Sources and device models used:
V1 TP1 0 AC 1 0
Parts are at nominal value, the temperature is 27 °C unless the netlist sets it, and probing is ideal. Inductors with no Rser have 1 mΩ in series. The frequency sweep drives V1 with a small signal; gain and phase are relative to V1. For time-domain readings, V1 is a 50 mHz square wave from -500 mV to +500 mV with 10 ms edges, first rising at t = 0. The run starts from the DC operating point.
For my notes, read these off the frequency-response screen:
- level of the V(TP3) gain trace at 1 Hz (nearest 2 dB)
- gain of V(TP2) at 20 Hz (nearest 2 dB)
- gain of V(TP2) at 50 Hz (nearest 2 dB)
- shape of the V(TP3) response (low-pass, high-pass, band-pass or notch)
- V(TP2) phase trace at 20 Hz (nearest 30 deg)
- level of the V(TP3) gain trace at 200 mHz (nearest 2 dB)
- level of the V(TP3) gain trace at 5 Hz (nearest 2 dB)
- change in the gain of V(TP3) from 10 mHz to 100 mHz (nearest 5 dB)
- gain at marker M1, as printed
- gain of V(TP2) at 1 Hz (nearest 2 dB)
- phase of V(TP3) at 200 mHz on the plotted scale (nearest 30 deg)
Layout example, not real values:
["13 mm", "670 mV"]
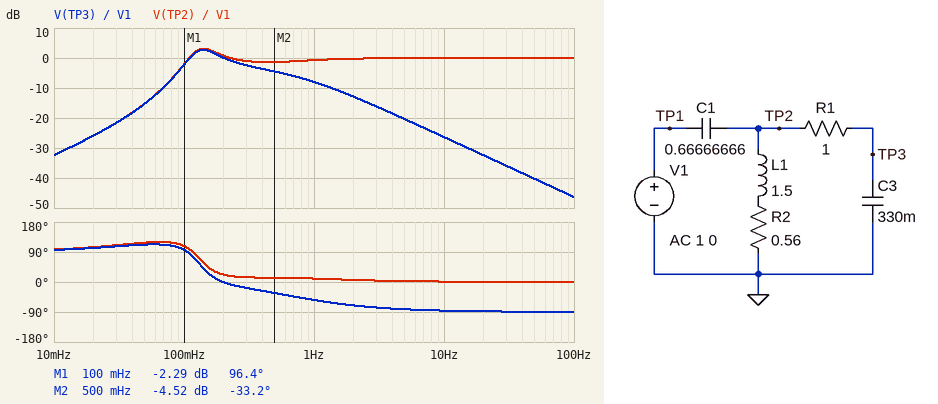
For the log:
["-8 dB", "0 dB", "0 dB", "band-pass", "0 deg", "0 dB", "-20 dB", "30 dB", "-2.29 dB", "0 dB", "0 deg"]
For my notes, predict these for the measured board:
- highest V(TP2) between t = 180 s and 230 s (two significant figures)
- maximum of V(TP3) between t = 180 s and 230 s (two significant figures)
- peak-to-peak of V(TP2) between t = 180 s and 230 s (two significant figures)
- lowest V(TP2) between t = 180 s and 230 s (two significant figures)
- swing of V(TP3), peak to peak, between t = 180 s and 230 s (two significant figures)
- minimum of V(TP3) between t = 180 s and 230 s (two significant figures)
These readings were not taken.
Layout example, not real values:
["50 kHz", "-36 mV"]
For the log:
["980 mV", "580 mV", "2.0 V", "-980 mV", "1.2 V", "-580 mV"]
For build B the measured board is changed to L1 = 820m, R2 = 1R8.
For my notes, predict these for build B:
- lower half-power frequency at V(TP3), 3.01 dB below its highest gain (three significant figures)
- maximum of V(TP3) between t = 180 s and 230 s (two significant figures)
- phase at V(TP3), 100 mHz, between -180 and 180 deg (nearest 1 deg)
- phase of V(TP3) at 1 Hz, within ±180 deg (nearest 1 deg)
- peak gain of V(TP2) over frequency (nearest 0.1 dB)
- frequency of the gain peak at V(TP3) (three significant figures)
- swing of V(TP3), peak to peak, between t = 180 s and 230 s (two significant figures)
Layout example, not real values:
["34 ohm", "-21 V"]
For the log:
["80.8 mHz", "560 mV", "38 deg", "-53 deg", "0 dB", "229 mHz", "1.1 V"]
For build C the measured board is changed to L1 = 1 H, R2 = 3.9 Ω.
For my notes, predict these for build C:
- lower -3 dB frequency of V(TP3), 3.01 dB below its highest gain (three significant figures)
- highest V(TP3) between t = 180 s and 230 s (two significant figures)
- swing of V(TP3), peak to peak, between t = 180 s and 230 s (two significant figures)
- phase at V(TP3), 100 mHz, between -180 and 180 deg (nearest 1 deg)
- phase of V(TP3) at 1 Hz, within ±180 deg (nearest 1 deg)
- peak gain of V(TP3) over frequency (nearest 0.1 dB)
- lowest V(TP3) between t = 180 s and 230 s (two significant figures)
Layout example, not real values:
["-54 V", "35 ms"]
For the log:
["38.3 mHz", "540 mV", "1.1 V", "15 deg", "-53 deg", "-3.6 dB", "-540 mV"]
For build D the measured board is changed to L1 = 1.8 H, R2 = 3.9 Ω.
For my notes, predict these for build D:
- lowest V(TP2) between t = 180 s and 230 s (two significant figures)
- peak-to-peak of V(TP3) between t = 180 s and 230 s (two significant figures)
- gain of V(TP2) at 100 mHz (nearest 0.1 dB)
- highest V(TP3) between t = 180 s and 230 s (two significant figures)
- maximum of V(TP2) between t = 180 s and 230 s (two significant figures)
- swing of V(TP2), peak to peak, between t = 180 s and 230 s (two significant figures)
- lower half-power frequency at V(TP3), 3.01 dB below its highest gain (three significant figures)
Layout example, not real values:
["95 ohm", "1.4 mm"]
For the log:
["-950 mV", "1.1 V", "-3.3 dB", "560 mV", "950 mV", "1.9 V", "39.5 mHz"]
